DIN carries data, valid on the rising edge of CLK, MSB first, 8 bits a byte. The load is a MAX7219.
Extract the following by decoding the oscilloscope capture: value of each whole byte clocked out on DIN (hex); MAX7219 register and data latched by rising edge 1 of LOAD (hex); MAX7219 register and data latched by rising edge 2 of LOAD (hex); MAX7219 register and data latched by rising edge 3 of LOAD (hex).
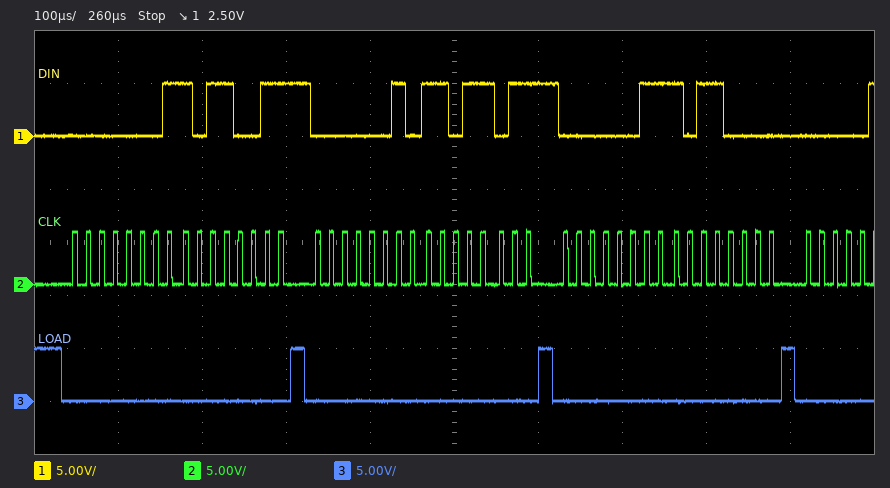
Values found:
0x01 0xB3 0x02 0xDB 0x03 0xB0
register 0x1, data 0xB3
register 0x2, data 0xDB
register 0x3, data 0xB0
